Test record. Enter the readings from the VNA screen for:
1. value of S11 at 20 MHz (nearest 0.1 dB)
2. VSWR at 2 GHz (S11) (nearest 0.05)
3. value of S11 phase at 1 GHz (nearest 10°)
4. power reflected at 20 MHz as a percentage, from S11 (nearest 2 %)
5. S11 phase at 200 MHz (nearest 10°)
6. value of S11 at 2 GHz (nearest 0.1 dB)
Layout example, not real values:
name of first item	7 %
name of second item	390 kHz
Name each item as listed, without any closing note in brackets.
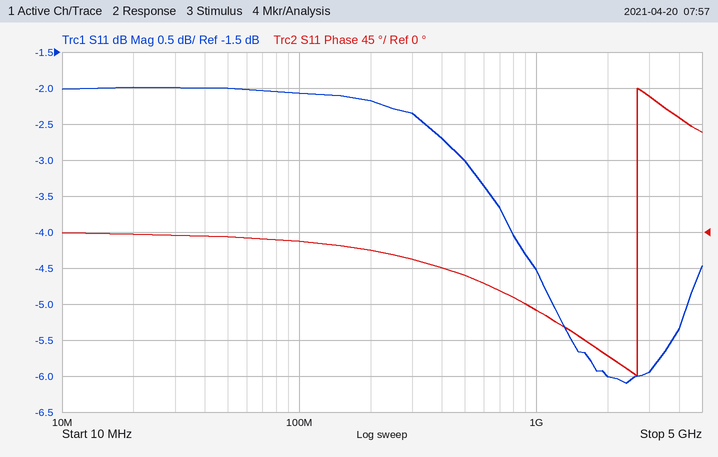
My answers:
value of S11 at 20 MHz	-2.0 dB
VSWR at 2 GHz (S11)	3.00
value of S11 phase at 1 GHz	-100°
power reflected at 20 MHz as a percentage, from S11	64 %
S11 phase at 200 MHz	-20°
value of S11 at 2 GHz	-6.0 dB
